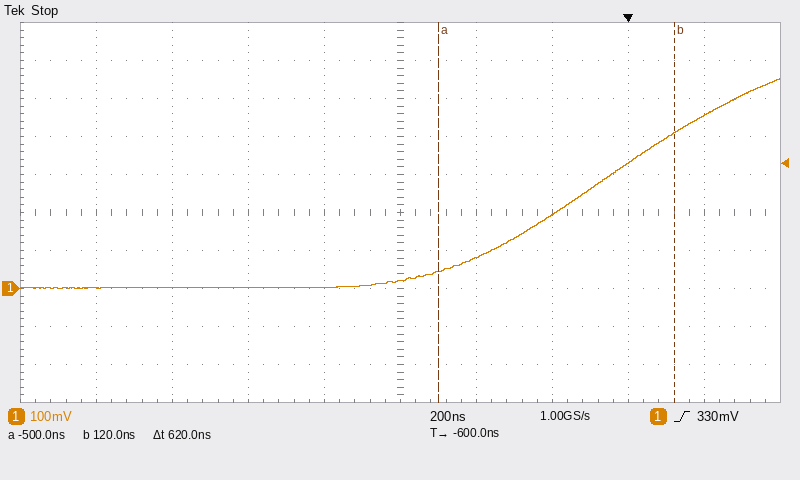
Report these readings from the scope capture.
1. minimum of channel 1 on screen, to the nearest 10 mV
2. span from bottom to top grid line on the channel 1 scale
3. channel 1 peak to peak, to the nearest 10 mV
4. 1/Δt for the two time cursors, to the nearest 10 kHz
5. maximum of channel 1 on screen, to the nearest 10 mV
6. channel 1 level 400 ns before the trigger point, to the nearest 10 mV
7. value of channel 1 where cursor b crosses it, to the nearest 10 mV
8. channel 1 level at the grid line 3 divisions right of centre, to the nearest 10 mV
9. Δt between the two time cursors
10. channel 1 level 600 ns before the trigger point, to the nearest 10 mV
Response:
0 mV
1 V
550 mV
1.61 MHz
550 mV
80 mV
410 mV
330 mV
620 ns
20 mV
